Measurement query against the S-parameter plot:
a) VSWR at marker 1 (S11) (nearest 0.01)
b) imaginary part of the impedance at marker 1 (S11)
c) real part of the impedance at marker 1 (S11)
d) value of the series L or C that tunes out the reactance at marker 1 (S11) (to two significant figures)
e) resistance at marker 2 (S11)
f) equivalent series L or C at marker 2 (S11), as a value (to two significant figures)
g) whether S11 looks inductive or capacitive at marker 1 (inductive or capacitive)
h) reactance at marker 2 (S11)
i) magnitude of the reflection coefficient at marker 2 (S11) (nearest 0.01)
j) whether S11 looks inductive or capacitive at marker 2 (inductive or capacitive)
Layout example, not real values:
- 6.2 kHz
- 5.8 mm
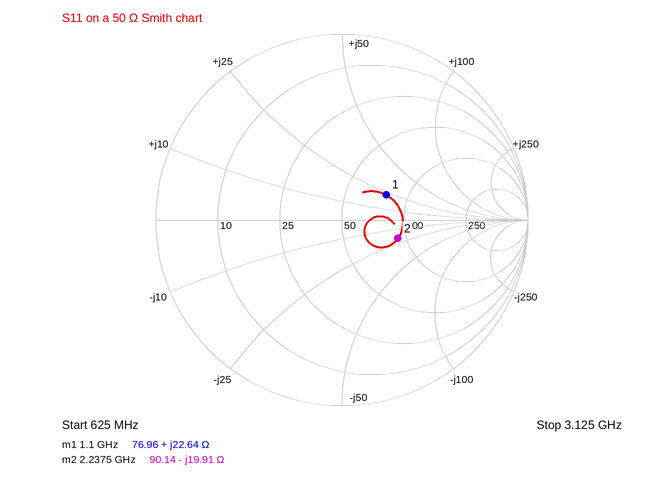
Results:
- 1.75
- +22.64 Ω
- 76.96 Ω
- 6.4 pF
- 90.14 Ω
- 3.6 pF
- inductive
- -19.91 Ω
- 0.32
- capacitive
